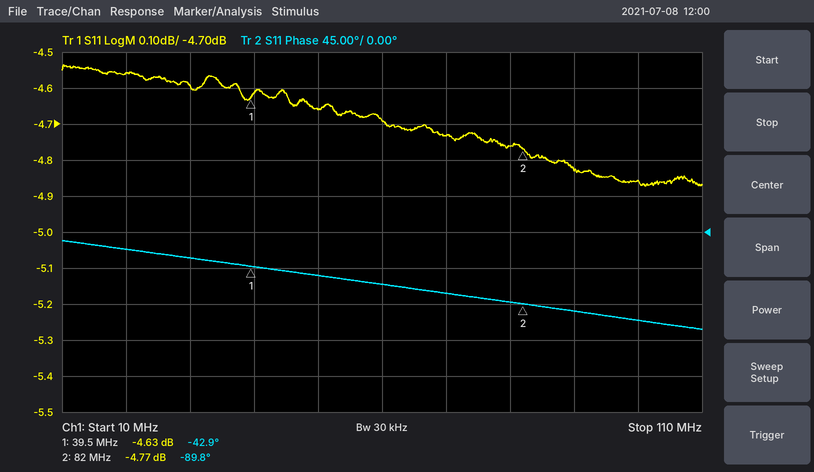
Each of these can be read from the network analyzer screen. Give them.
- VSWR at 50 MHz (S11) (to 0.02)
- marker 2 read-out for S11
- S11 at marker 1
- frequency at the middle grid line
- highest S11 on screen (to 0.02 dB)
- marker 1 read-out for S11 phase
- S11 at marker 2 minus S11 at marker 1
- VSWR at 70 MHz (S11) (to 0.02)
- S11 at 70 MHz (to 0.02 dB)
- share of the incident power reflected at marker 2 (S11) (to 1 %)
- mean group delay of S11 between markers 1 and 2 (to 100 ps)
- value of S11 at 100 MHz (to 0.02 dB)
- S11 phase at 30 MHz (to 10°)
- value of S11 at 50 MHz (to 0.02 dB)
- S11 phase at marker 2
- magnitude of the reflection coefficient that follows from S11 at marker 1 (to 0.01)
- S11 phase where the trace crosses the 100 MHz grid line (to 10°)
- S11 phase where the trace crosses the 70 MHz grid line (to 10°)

3.82
-4.77 dB
-4.63 dB
60 MHz
-4.54 dB
-42.9°
-0.14 dB
3.76
-4.74 dB
33 %
3.1 ns
-4.86 dB
-30°
-4.66 dB
-89.8°
0.59
-110°
-80°
